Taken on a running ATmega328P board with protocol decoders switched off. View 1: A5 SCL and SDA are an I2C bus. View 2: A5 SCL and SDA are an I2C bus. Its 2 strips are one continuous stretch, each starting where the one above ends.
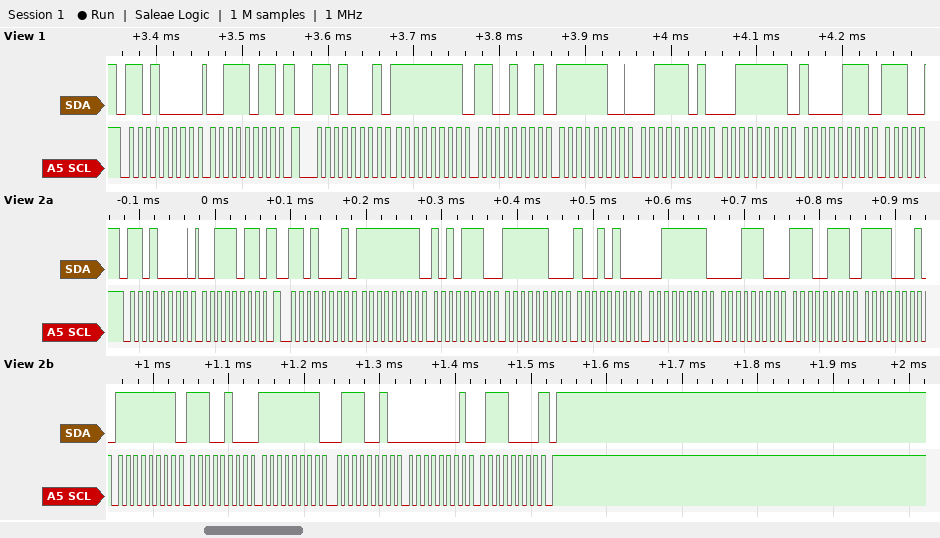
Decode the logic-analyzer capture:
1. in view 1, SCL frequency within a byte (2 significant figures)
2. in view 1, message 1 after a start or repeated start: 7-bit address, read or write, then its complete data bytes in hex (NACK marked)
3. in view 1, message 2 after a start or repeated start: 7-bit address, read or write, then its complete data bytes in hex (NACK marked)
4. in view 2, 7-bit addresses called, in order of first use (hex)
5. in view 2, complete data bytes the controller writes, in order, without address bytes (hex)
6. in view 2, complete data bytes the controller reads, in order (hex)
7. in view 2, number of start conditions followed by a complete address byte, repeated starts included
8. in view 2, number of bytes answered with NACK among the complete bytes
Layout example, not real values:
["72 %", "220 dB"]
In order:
["100 kHz", "0x68 write: 3B", "0x68 read: FF C9 FC 3D 3F 87", "0x68", "3B", "FF AE FC 94 3F 1C E7 F1 FF E4 FF 72 01 70", "2", "1"]
